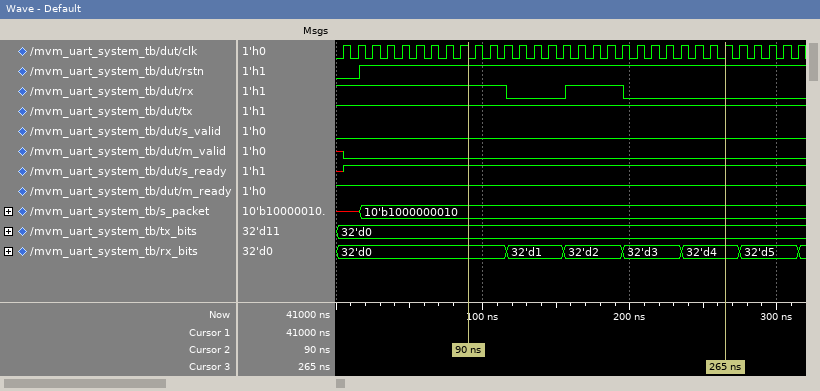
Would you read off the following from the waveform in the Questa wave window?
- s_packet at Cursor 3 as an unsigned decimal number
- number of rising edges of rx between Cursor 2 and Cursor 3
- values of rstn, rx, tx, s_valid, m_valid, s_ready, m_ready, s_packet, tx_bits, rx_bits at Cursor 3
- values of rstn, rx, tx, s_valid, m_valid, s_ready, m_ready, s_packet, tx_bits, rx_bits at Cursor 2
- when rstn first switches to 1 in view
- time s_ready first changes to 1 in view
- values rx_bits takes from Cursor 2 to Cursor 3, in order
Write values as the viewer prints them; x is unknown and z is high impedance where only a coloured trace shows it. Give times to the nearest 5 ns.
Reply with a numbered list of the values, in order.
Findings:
1. 514
2. 1
3. rstn=1, rx=0, tx=1, s_valid=0, m_valid=0, s_ready=1, m_ready=1, s_packet=10'b1000000010, tx_bits=32'd0, rx_bits=32'd4
4. rstn=1, rx=1, tx=1, s_valid=0, m_valid=0, s_ready=1, m_ready=1, s_packet=10'b1000000010, tx_bits=32'd0, rx_bits=32'd0
5. 15 ns
6. 5 ns
7. 32'd0, 32'd1, 32'd2, 32'd3, 32'd4
